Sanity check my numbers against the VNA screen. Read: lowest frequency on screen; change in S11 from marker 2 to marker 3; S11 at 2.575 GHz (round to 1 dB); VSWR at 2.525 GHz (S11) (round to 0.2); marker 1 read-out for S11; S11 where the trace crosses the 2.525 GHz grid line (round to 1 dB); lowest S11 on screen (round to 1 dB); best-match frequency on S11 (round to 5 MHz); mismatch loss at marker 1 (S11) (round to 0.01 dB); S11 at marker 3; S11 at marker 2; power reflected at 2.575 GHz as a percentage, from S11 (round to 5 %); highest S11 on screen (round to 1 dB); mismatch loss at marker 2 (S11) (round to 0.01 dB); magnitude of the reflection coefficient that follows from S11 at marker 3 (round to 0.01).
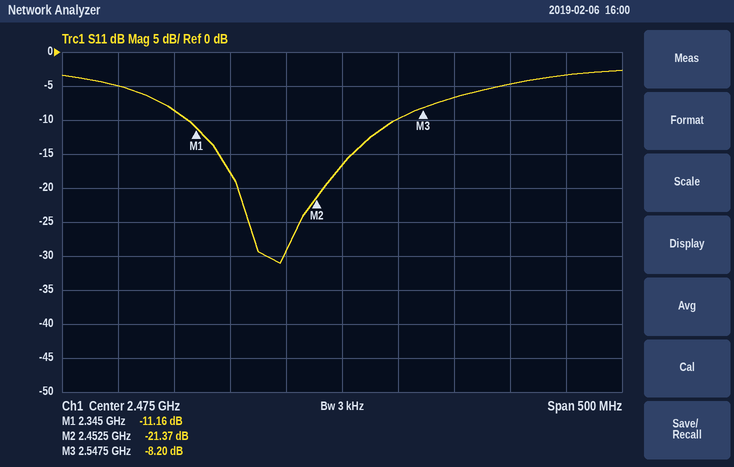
2.225 GHz
13.17 dB
-7 dB
2.0
-11.16 dB
-10 dB
-31 dB
2.420 GHz
0.35 dB
-8.20 dB
-21.37 dB
20 %
-3 dB
0.03 dB
0.39
